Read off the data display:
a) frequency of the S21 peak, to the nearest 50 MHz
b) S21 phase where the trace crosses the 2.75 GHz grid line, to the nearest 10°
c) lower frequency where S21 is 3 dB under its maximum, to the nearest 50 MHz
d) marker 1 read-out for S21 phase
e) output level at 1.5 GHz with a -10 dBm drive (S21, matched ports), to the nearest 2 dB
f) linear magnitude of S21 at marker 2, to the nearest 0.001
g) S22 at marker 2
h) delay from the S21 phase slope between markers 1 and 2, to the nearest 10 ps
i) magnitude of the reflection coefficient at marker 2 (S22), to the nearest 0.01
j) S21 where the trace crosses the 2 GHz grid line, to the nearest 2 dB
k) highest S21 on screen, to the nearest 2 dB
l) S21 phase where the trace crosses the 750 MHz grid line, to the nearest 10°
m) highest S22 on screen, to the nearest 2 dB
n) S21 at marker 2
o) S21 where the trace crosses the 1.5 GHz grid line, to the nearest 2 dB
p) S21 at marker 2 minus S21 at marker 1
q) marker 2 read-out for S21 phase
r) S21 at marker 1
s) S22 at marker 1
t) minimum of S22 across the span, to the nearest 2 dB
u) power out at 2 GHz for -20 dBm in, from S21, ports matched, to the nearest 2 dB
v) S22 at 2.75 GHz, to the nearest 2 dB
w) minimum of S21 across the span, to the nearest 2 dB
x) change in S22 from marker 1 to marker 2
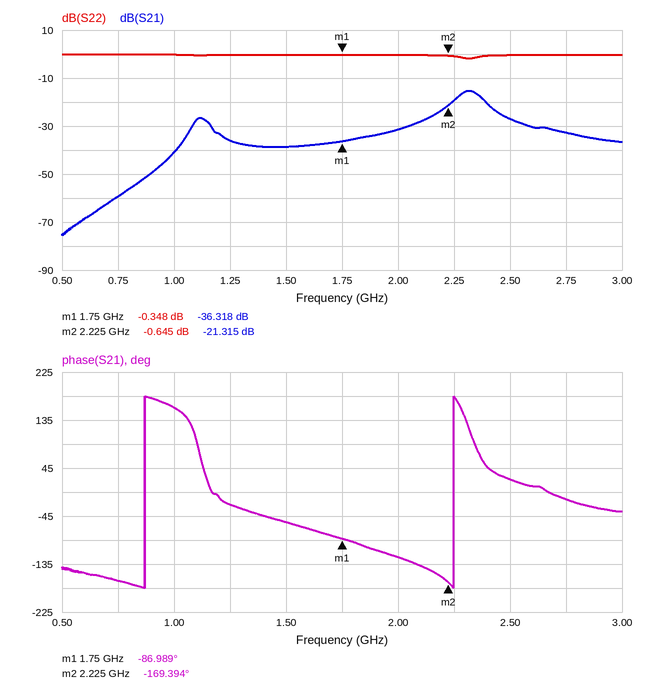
2.30 GHz
-10°
2.25 GHz
-86.989°
-48 dBm
0.086
-0.645 dB
480 ps
0.93
-32 dB
-16 dB
-170°
0 dB
-21.315 dB
-38 dB
15.003 dB
-169.394°
-36.318 dB
-0.348 dB
-2 dB
-52 dBm
0 dB
-76 dB
-0.297 dB
